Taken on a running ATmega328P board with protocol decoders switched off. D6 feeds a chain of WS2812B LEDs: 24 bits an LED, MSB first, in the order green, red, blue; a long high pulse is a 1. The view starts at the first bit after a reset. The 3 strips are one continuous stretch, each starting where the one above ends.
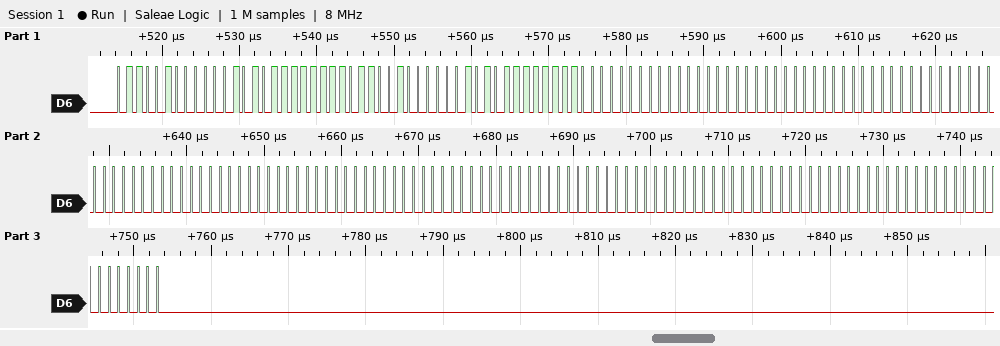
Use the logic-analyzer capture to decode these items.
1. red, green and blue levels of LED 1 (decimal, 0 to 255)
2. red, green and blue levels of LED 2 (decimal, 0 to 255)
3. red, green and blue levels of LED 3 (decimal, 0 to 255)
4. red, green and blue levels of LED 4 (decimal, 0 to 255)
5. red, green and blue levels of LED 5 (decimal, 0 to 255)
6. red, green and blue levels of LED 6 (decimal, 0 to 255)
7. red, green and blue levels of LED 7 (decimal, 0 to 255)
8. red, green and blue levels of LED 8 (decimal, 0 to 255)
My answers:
10, 100, 255
10, 100, 255
0, 0, 0
0, 0, 0
0, 0, 0
0, 0, 0
0, 0, 0
0, 0, 0
